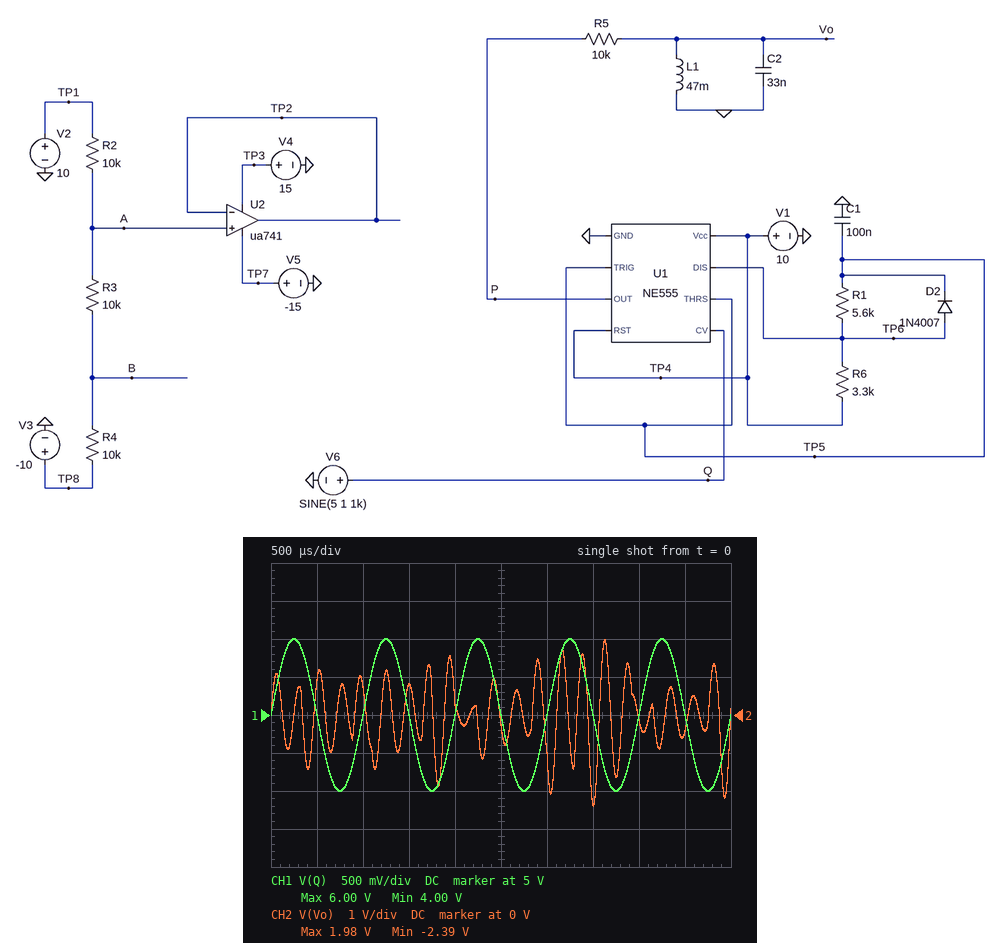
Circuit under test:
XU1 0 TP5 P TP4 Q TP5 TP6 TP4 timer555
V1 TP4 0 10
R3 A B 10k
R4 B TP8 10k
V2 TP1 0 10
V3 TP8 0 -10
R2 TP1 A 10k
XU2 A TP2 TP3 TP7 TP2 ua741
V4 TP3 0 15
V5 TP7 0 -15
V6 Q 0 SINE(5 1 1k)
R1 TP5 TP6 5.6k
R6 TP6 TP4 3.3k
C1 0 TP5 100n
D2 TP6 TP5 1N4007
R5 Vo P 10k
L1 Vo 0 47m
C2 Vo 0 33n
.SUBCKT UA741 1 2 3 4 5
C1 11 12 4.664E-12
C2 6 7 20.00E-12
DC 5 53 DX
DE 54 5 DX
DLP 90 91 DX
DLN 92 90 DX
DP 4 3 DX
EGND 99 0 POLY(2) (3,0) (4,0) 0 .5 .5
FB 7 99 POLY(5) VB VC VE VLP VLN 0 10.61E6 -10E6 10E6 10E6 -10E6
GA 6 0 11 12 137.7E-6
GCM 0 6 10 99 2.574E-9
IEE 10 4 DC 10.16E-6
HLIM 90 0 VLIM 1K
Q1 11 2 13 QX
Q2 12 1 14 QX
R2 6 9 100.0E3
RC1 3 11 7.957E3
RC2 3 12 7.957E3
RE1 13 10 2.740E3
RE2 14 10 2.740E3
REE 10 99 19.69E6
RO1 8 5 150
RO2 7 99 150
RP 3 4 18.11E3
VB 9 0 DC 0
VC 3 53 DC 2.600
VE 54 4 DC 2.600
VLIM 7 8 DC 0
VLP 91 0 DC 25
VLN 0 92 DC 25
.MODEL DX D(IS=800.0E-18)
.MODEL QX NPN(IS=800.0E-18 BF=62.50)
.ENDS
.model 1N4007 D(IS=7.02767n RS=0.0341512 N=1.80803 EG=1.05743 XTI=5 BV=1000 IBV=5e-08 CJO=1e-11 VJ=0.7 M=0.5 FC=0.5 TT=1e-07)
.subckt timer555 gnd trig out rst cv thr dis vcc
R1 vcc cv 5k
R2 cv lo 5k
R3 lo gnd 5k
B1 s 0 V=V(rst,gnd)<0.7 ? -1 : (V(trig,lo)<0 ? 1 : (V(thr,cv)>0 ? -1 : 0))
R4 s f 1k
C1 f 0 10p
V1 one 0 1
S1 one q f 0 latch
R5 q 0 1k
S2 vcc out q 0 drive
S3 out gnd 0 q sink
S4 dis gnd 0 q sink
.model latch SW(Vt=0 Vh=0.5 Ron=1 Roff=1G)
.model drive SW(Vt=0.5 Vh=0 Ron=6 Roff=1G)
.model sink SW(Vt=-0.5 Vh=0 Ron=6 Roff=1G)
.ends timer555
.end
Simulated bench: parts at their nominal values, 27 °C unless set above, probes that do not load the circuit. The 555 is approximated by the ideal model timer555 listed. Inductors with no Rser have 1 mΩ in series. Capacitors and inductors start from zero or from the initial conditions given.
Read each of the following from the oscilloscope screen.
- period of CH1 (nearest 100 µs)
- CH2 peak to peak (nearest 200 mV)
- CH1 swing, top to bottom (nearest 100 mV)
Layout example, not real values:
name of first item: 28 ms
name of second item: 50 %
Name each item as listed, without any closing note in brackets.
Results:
period of CH1: 1.0 ms
CH2 peak to peak: 4.4 V
CH1 swing, top to bottom: 2.0 V
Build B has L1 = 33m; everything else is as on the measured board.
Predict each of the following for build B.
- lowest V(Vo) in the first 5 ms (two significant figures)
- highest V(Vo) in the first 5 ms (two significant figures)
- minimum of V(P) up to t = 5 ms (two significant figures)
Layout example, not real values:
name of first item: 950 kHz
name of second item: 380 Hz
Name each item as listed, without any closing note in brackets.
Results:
lowest V(Vo) in the first 5 ms: -1.9 V
highest V(Vo) in the first 5 ms: 1.7 V
minimum of V(P) up to t = 5 ms: -1.1 mV
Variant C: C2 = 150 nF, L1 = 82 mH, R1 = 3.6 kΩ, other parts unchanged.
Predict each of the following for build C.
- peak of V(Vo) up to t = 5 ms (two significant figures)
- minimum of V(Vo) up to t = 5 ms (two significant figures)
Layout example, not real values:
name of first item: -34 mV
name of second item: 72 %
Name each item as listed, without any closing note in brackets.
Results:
peak of V(Vo) up to t = 5 ms: 1.7 V
minimum of V(Vo) up to t = 5 ms: -1.3 V
